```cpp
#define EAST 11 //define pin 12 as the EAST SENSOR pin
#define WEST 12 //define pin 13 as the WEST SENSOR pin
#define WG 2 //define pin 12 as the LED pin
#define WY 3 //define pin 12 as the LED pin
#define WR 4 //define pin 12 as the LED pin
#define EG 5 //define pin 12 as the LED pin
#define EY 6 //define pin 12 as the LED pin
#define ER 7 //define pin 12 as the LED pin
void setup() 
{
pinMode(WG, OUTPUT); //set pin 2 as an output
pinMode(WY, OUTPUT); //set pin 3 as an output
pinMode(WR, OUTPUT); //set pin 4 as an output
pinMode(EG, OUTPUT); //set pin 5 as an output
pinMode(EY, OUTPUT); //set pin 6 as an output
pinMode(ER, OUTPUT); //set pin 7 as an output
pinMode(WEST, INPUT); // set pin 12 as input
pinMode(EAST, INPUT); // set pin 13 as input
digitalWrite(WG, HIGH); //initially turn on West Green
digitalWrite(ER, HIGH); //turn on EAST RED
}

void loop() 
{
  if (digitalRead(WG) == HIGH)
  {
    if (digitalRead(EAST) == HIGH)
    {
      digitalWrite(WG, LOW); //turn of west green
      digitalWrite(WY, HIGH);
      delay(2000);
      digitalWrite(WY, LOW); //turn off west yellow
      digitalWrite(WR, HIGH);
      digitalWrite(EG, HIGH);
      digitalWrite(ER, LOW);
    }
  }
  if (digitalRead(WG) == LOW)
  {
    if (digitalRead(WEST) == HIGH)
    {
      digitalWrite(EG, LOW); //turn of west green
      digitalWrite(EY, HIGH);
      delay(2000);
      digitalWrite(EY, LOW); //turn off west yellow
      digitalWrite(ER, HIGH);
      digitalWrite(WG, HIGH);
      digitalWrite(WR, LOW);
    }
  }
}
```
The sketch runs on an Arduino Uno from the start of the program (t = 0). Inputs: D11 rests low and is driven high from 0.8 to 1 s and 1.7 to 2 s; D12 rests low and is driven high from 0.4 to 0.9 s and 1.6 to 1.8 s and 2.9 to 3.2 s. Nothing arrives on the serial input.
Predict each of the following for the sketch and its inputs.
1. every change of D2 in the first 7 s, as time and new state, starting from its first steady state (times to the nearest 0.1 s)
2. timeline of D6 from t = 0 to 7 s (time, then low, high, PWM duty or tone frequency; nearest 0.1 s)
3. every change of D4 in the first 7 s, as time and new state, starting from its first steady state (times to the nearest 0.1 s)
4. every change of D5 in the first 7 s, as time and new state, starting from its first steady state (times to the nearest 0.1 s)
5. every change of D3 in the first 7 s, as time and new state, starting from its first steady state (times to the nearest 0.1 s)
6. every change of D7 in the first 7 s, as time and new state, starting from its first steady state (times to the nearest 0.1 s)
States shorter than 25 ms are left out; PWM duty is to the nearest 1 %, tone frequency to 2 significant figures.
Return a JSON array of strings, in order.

["0 s high; 0.8 s low; 4.9 s high", "0 s low; 2.9 s high; 4.9 s low", "0 s low; 2.8 s high; 4.9 s low", "0 s low; 2.8 s high; 2.9 s low", "0 s low; 0.8 s high; 2.8 s low", "0 s high; 2.8 s low; 4.9 s high"]
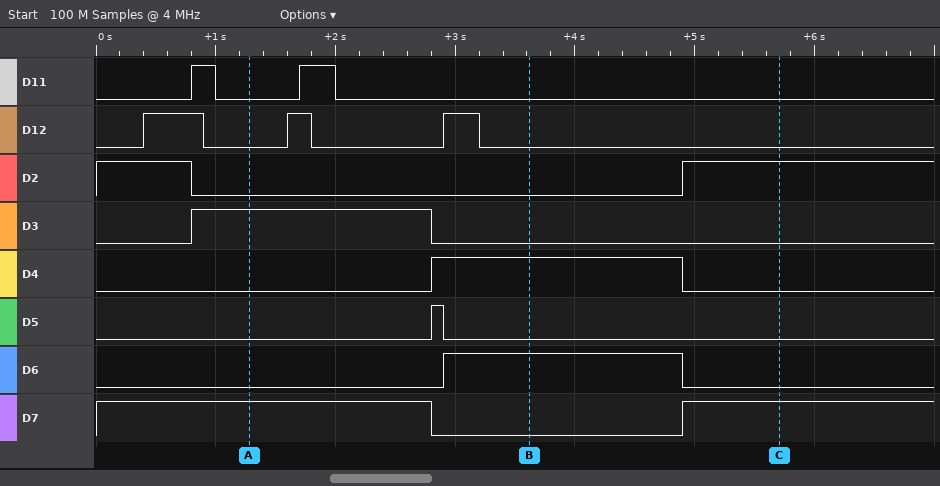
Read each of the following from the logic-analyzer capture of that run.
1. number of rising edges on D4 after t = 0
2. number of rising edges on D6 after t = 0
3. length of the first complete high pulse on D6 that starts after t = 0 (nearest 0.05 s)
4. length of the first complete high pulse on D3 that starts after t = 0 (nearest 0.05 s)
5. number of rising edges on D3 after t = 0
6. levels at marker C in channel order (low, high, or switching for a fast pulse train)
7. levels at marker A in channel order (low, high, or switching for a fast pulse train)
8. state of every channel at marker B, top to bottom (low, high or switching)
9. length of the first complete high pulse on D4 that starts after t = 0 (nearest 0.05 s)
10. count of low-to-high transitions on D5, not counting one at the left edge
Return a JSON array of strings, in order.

["1", "1", "2.00 s", "2.00 s", "1", "D11 low, D12 low, D2 high, D3 low, D4 low, D5 low, D6 low, D7 high", "D11 low, D12 low, D2 low, D3 high, D4 low, D5 low, D6 low, D7 high", "D11 low, D12 low, D2 low, D3 low, D4 high, D5 low, D6 high, D7 low", "2.10 s", "1"]
